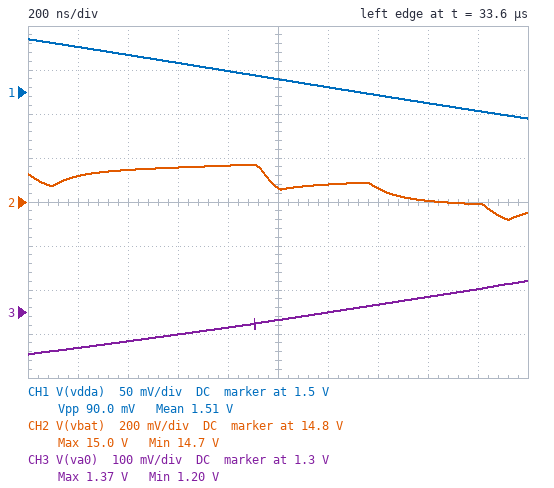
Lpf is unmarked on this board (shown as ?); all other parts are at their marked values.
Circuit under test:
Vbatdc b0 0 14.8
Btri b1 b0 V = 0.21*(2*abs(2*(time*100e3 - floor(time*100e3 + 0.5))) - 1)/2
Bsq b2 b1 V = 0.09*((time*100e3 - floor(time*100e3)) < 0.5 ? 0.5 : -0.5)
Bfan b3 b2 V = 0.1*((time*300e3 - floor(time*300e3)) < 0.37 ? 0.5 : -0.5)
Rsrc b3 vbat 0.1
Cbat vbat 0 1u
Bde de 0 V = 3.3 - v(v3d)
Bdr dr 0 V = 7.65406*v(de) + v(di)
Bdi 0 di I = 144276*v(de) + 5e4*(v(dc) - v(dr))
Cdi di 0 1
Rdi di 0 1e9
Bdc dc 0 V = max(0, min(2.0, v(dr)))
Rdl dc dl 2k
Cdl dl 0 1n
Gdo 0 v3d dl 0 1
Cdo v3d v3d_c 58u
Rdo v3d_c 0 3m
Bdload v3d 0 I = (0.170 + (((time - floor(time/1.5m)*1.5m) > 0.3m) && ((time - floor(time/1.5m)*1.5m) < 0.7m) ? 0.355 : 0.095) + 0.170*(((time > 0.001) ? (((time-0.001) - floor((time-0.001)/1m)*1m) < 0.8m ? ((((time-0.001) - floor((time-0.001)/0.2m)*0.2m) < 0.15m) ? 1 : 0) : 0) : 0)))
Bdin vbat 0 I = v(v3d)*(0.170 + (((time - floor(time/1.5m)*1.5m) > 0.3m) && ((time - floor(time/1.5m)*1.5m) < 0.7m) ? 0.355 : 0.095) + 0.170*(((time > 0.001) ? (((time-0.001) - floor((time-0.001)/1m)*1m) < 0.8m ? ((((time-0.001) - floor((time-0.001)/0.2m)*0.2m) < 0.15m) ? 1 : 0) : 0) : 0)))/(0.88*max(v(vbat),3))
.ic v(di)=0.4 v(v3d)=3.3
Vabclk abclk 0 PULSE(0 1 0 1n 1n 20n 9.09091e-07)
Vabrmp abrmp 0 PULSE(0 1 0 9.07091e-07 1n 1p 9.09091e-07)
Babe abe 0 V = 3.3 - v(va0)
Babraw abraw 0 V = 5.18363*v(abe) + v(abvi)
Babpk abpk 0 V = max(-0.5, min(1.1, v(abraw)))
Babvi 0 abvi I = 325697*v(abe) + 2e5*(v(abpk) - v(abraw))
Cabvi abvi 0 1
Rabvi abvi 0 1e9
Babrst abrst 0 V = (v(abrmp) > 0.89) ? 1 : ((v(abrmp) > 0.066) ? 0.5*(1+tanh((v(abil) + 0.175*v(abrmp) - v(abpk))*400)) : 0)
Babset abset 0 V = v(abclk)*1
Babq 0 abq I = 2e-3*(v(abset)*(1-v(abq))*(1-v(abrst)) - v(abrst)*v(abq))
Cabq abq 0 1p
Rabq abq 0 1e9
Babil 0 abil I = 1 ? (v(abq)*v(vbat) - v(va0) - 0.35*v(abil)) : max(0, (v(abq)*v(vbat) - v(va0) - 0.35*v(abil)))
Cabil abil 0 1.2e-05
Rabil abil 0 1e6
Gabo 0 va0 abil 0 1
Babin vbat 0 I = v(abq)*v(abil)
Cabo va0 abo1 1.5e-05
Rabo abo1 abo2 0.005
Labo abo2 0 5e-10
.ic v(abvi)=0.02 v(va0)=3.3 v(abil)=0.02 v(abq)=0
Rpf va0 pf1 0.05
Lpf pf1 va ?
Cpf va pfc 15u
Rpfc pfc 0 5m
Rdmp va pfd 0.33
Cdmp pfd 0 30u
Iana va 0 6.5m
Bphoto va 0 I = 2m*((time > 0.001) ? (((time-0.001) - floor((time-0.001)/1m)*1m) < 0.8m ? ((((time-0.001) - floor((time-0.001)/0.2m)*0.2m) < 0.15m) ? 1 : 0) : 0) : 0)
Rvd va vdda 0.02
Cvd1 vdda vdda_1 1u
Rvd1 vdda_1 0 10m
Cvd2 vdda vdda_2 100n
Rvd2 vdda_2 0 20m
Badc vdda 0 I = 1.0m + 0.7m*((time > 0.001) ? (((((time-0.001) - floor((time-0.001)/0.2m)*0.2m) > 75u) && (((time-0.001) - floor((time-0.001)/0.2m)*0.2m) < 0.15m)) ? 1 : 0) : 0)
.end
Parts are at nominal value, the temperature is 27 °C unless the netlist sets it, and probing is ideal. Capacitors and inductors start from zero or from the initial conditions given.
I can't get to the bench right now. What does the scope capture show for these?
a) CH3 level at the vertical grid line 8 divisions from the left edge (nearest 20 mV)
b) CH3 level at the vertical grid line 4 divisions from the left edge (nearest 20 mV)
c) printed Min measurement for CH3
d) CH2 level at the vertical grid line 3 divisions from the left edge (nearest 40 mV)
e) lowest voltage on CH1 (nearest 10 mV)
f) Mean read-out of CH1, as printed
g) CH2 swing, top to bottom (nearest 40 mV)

1.34 V
1.26 V
1.20 V
14.96 V
1.47 V
1.51 V
240 mV
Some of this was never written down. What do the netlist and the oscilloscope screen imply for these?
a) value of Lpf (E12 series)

1.2 µH
